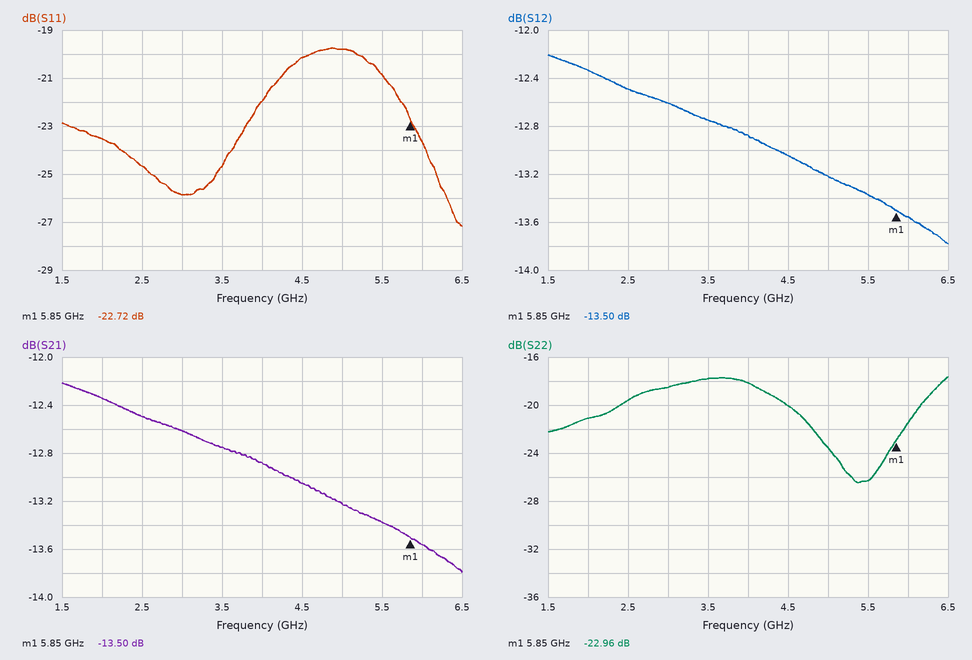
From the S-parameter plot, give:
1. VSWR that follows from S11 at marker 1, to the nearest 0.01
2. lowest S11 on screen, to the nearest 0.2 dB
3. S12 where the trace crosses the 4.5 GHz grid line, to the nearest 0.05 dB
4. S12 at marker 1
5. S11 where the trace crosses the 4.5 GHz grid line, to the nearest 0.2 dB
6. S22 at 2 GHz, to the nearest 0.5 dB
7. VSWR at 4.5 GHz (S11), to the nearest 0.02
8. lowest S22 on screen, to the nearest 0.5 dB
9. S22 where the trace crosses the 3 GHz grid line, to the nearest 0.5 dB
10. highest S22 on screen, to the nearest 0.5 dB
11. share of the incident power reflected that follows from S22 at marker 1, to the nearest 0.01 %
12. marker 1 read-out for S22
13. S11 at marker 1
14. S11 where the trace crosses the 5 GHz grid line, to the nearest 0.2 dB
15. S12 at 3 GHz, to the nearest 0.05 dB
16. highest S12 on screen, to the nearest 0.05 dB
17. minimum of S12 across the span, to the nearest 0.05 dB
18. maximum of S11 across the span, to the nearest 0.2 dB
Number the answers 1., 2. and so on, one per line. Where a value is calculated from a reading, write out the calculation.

1. (1 + 0.0731)/(1 − 0.0731) ≈ 1.16
2. -27.2 dB
3. -13.05 dB
4. -13.50 dB
5. -20.2 dB
6. -21.0 dB
7. |Γ| = 10^(-20.2/20) = 0.0977; VSWR = (1 + 0.0977)/(1 − 0.0977) ≈ 1.22
8. -26.5 dB
9. -18.5 dB
10. -17.5 dB
11. 10^(-22.96/10) ≈ 0.51 %
12. -22.96 dB
13. -22.72 dB
14. -19.8 dB
15. -12.60 dB
16. -12.20 dB
17. -13.80 dB
18. -19.8 dB
